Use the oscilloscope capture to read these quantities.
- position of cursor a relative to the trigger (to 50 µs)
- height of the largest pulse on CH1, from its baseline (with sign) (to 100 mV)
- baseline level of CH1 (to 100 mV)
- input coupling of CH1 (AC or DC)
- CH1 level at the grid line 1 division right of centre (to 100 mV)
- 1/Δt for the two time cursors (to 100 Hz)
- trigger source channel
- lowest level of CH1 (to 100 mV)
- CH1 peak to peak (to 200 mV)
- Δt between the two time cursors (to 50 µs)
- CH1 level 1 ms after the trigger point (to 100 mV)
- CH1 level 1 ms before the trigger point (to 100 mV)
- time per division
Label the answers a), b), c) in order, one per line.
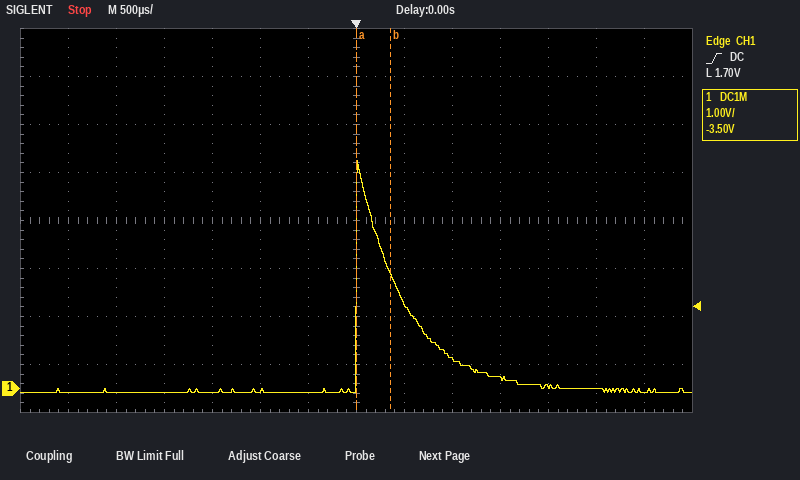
a) 0 µs
b) +4.8 V
c) -100 mV
d) DC
e) 1.8 V
f) 2.9 kHz
g) CH1
h) -100 mV
i) 4.8 V
j) 350 µs
k) 600 mV
l) 0.0 V
m) 500 µs
